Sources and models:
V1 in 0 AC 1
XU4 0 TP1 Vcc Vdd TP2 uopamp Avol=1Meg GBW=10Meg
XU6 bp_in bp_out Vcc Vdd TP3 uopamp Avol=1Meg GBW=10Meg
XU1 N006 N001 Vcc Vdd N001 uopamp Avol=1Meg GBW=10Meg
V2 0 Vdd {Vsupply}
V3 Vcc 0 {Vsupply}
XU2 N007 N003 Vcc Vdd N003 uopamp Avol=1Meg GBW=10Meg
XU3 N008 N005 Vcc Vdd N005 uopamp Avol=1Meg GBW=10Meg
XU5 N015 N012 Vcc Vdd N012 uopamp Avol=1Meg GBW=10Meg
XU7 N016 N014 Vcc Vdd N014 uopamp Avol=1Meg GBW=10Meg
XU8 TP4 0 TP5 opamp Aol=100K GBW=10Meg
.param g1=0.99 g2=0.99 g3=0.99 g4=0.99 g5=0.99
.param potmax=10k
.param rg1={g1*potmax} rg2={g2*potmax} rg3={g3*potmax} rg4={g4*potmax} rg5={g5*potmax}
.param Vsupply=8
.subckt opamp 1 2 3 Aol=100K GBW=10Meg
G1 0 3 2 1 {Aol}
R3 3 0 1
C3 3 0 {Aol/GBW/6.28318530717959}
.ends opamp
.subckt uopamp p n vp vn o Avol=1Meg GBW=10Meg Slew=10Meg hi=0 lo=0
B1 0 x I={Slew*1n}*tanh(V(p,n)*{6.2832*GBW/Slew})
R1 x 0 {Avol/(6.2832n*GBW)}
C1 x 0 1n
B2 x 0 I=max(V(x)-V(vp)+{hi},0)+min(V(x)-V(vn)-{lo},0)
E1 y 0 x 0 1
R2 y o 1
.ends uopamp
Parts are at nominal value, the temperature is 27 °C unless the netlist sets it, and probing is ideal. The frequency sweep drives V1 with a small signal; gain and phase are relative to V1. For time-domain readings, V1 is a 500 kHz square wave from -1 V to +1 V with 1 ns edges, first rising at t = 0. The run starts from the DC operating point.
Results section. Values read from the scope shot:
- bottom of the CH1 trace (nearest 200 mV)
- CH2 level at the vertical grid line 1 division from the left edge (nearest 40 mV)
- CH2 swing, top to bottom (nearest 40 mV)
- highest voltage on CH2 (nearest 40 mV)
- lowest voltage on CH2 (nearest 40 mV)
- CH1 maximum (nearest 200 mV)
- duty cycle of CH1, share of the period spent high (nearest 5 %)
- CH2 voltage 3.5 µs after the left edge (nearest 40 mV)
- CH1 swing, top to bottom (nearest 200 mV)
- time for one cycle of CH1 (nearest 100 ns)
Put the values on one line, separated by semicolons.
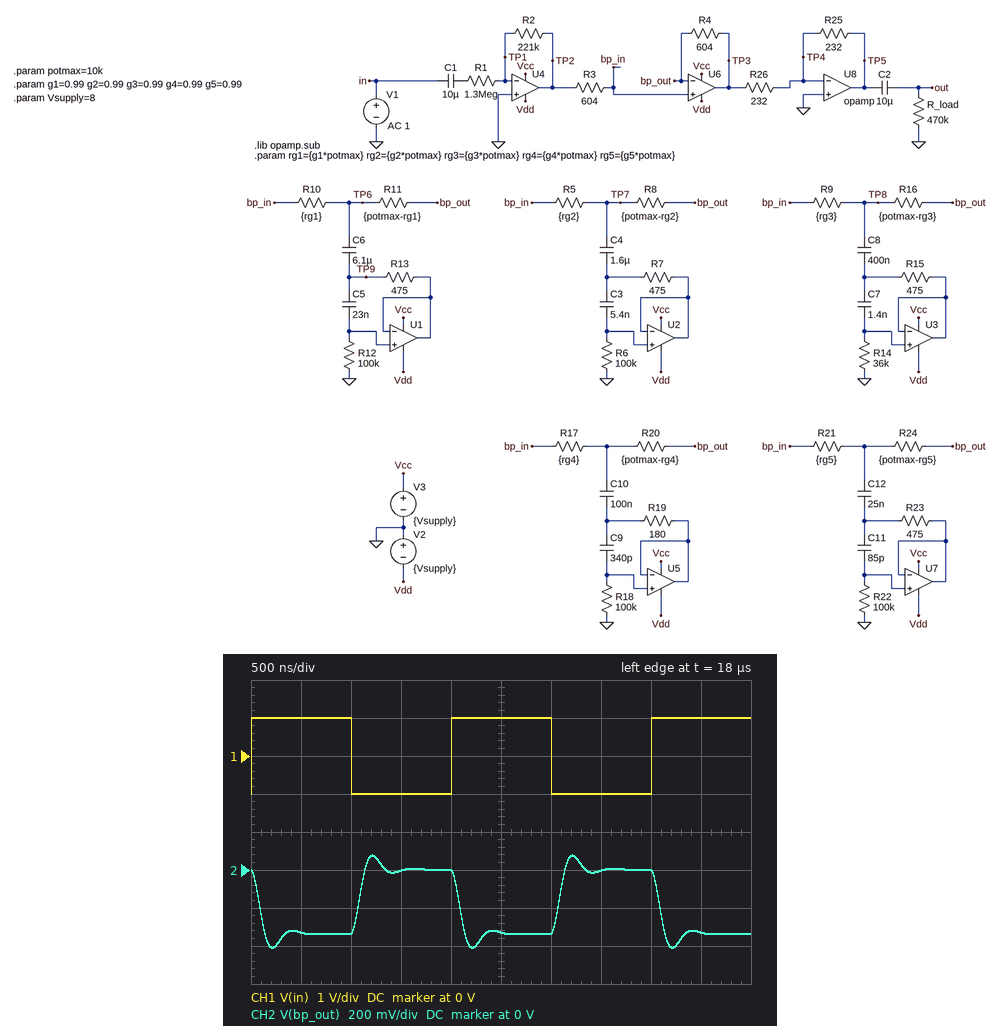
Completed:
-1.0 V; -320 mV; 480 mV; 80 mV; -400 mV; 1.0 V; 50 %; 0 V; 2.0 V; 2.0 µs
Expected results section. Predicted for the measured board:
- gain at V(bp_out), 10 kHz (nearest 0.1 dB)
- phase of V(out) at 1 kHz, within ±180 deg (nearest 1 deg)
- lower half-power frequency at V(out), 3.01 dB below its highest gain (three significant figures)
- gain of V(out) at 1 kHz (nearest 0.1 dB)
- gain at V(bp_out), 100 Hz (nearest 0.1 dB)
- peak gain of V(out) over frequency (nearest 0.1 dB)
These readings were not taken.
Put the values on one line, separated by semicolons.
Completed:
-15.6 dB; 11 deg; 2.99 kHz; -8.9 dB; -15.5 dB; -4.0 dB
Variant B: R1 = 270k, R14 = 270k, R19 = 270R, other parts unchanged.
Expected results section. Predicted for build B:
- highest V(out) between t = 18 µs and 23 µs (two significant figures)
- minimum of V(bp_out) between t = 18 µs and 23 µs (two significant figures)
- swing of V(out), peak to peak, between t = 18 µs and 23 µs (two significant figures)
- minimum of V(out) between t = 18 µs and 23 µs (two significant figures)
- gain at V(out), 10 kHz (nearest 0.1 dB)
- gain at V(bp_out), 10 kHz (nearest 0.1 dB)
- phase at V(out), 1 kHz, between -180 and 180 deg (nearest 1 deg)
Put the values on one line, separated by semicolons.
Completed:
3.5 V; -1.8 V; 3.0 V; 480 mV; 6.0 dB; -1.9 dB; -16 deg
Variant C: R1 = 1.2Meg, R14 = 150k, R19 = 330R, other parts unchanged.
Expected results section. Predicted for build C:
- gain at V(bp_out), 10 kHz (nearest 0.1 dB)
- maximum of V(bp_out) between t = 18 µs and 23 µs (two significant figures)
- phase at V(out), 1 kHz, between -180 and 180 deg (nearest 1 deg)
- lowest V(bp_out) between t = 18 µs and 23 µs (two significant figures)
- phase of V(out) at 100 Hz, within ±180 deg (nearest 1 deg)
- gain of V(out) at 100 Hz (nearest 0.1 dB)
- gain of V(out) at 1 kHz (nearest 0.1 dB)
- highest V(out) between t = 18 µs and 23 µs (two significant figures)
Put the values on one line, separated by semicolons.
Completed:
-14.8 dB; 74 mV; -8 deg; -440 mV; 5 deg; -8.6 dB; -8.0 dB; 870 mV
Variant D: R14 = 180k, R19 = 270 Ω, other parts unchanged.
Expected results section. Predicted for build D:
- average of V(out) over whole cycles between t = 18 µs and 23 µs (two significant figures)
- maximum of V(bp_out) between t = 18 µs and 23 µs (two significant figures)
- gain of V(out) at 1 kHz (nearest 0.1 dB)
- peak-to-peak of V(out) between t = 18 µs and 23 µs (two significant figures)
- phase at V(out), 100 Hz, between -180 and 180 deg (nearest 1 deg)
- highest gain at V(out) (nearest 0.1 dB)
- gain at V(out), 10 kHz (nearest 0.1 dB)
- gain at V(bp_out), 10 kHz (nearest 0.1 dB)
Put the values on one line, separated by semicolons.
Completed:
420 mV; 71 mV; -9.3 dB; 840 mV; 5 deg; -6.3 dB; -7.6 dB; -15.5 dB
